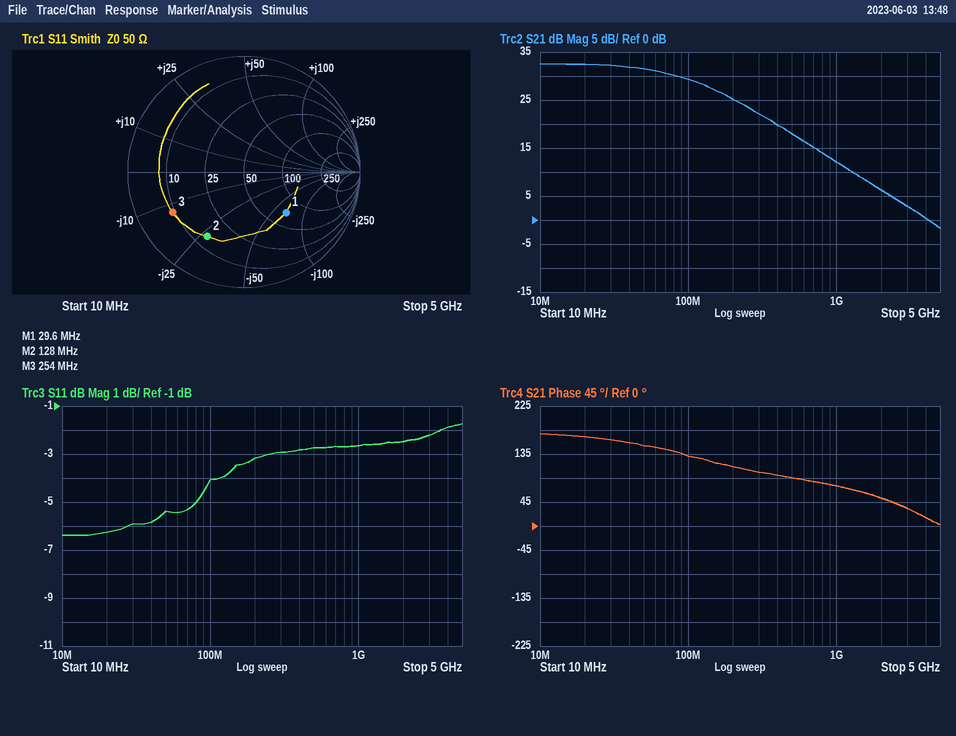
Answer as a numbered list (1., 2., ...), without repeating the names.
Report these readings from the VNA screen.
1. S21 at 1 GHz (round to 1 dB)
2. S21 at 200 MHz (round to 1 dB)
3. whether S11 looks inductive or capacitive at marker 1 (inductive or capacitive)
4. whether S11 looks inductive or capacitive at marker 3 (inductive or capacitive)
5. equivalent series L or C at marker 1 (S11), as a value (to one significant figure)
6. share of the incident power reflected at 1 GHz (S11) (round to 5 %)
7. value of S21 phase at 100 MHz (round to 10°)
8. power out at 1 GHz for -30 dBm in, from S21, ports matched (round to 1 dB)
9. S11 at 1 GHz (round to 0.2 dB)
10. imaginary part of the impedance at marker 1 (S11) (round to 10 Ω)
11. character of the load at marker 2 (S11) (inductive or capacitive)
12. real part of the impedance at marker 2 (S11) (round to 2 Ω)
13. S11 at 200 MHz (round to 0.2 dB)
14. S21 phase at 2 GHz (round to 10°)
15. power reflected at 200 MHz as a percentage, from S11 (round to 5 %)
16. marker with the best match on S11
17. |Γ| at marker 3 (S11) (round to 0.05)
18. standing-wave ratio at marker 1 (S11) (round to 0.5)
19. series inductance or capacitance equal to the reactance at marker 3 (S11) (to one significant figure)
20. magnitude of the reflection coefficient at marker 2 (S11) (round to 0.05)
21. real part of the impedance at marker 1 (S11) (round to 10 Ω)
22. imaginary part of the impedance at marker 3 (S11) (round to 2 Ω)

1. 12 dB
2. 25 dB
3. capacitive
4. capacitive
5. 80 pF
6. 55 %
7. 130°
8. -18 dBm
9. -2.6 dB
10. -70 Ω
11. capacitive
12. 14 Ω
13. -3.2 dB
14. 50°
15. 50 %
16. marker 1
17. 0.70
18. 3.0
19. 50 pF
20. 0.65
21. 70 Ω
22. -12 Ω
